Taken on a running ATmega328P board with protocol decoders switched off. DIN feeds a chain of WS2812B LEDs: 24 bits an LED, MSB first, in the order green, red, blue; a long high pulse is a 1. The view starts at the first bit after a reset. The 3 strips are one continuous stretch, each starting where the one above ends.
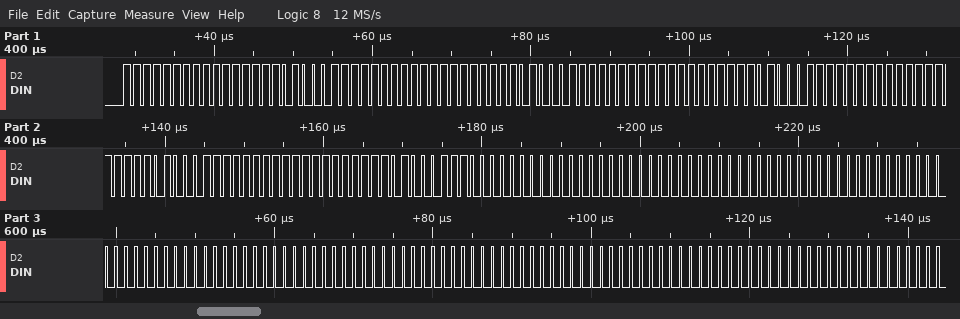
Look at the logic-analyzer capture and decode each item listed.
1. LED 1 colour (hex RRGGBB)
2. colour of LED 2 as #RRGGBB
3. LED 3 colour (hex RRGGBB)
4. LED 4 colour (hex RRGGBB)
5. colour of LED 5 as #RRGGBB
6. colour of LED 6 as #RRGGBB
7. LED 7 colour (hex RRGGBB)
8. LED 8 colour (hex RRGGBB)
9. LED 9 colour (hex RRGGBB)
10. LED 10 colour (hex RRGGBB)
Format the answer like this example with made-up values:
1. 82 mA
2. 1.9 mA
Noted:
1. #FFFF47
2. #FFFF47
3. #FFFF47
4. #FFFF47
5. #FFFF47
6. #000000
7. #000000
8. #000000
9. #000000
10. #000000
